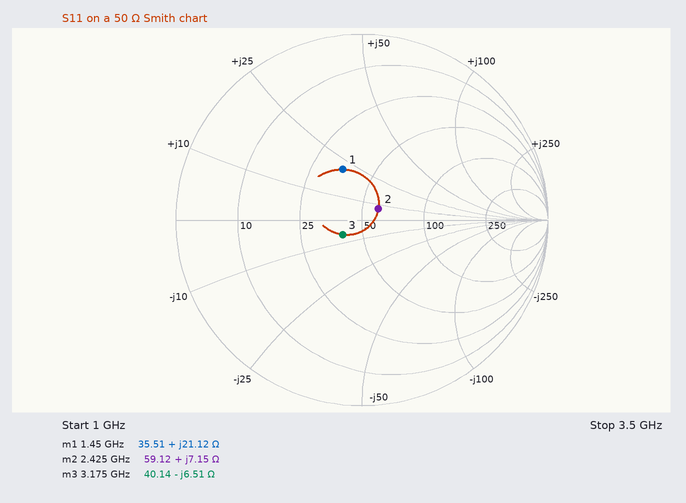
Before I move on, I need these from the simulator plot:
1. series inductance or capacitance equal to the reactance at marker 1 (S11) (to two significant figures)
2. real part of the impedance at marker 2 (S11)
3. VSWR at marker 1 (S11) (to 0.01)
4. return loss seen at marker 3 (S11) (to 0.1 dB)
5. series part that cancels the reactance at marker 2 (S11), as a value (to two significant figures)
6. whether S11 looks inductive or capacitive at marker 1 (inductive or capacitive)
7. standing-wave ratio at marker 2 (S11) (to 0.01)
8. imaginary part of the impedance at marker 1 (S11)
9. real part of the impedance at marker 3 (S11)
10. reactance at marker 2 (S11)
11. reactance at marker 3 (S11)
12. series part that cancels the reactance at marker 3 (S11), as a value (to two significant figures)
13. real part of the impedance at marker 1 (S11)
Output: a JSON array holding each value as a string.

["2.3 nH", "59.12 Ω", "1.82", "17.7 dB", "9.2 pF", "inductive", "1.24", "+21.12 Ω", "40.14 Ω", "+7.15 Ω", "-6.51 Ω", "330 pH", "35.51 Ω"]
